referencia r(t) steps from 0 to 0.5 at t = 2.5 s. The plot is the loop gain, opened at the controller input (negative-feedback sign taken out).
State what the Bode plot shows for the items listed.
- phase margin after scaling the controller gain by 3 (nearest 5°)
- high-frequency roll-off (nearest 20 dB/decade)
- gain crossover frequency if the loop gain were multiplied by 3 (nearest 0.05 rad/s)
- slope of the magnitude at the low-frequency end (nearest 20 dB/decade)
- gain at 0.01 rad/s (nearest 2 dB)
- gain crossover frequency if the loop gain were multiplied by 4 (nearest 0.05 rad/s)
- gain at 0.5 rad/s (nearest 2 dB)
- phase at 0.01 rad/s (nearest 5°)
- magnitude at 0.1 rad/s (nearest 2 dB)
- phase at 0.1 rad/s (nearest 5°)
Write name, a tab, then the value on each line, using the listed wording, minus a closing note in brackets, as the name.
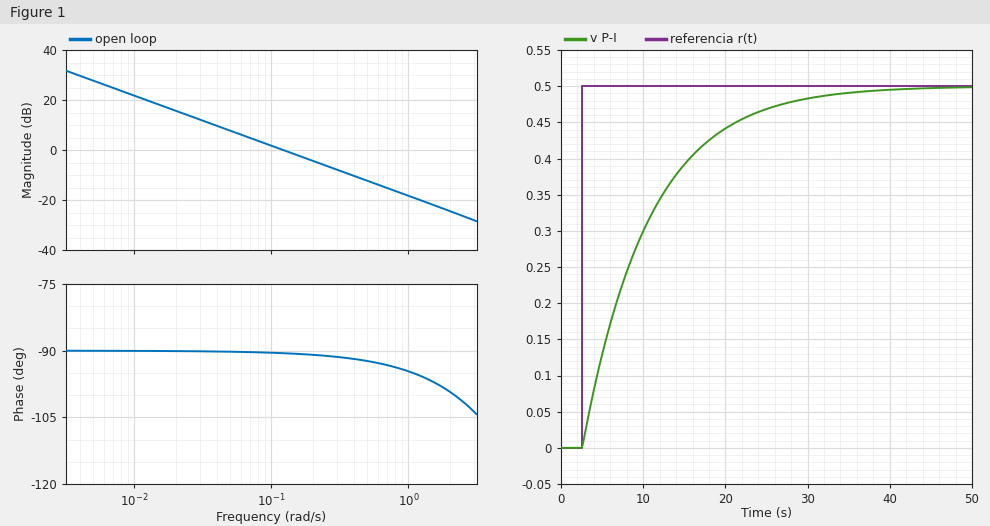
phase margin after scaling the controller gain by 3	90°
high-frequency roll-off	-20 dB/decade
gain crossover frequency if the loop gain were multiplied by 3	0.35 rad/s
slope of the magnitude at the low-frequency end	-20 dB/decade
gain at 0.01 rad/s	22 dB
gain crossover frequency if the loop gain were multiplied by 4	0.50 rad/s
gain at 0.5 rad/s	-12 dB
phase at 0.01 rad/s	-90°
magnitude at 0.1 rad/s	2 dB
phase at 0.1 rad/s	-90°
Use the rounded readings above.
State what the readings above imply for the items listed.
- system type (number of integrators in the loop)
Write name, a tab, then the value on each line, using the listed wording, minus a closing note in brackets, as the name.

system type	1
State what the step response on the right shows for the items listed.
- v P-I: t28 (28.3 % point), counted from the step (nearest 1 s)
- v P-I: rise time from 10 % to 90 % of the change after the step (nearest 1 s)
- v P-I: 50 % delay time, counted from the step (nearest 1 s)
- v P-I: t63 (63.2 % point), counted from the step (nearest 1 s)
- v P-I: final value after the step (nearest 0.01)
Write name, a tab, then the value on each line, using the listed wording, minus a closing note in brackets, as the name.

v P-I: t28 (28.3 % point), counted from the step	3 s
v P-I: rise time from 10 % to 90 % of the change after the step	18 s
v P-I: 50 % delay time, counted from the step	6 s
v P-I: t63 (63.2 % point), counted from the step	8 s
v P-I: final value after the step	0.50
